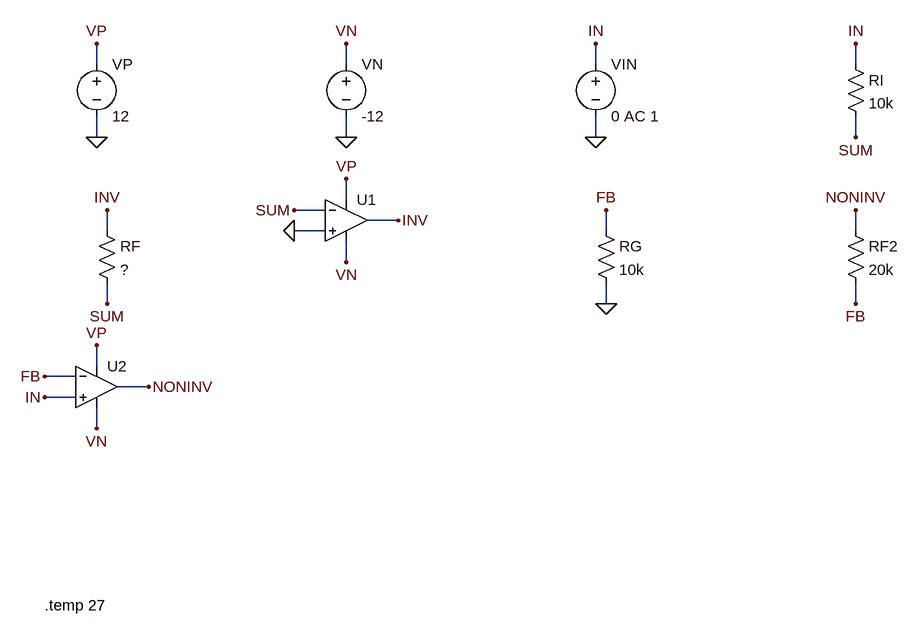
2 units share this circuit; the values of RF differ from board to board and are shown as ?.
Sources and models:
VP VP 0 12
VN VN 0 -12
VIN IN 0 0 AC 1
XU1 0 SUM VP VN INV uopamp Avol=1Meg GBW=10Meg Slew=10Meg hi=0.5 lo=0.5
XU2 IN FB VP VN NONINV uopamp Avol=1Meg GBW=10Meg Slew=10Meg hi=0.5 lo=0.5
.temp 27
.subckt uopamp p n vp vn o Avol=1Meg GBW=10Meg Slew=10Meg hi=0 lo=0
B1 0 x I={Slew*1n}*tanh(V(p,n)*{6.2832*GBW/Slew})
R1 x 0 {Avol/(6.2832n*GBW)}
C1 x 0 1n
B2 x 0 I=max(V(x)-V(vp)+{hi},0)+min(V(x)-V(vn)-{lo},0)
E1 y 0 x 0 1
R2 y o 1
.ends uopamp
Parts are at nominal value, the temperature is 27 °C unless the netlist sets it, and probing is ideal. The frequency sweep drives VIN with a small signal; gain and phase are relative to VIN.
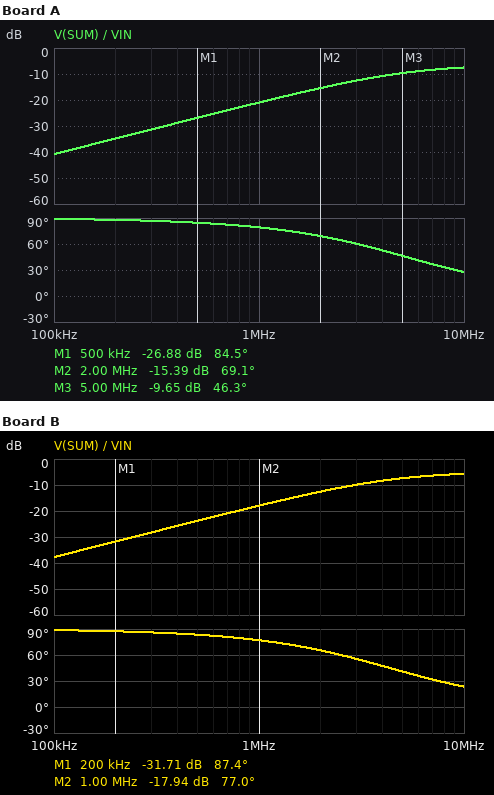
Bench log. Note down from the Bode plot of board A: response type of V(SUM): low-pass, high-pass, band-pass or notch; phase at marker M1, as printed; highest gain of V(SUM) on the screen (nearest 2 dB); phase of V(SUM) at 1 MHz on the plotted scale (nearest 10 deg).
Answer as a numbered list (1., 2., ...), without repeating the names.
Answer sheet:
1. high-pass
2. 84.5 deg
3. -8 dB
4. 80 deg
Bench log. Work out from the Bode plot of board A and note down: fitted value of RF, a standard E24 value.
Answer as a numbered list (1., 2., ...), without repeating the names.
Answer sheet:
1. 9.1 kΩ
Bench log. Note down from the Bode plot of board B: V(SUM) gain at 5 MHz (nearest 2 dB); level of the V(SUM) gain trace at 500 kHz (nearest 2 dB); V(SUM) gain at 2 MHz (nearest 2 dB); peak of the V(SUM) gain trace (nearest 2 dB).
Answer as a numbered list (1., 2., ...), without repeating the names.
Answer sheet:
1. -8 dB
2. -24 dB
3. -12 dB
4. -6 dB
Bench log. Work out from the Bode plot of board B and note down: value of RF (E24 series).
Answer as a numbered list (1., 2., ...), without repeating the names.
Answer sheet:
1. 13 kΩ
